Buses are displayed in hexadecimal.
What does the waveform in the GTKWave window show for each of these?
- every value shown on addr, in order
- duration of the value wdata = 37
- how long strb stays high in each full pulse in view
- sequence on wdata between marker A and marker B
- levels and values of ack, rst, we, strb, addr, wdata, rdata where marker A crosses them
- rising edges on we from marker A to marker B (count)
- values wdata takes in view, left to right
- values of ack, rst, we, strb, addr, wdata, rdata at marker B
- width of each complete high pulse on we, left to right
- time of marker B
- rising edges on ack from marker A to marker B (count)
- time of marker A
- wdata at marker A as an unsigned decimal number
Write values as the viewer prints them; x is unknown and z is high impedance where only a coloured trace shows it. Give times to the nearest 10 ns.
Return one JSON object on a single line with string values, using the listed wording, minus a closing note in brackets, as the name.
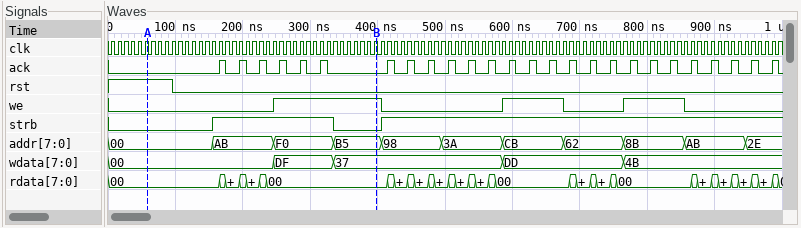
{"every value shown on addr, in order": "00, AB, F0, B5, 98, 3A, CB, 62, 8B, AB, 2E", "duration of the value wdata = 37": "250 ns", "how long strb stays high in each full pulse in view": "180 ns", "sequence on wdata between marker A and marker B": "00, DF, 37", "levels and values of ack, rst, we, strb, addr, wdata, rdata where marker A crosses them": "ack=0, rst=1, we=0, strb=0, addr=00, wdata=00, rdata=00", "rising edges on we from marker A to marker B": "1", "values wdata takes in view, left to right": "00, DF, 37, DD, 4B", "values of ack, rst, we, strb, addr, wdata, rdata at marker B": "ack=0, rst=0, we=1, strb=0, addr=B5, wdata=37, rdata=00", "width of each complete high pulse on we, left to right": "160 ns, 90 ns, 90 ns", "time of marker B": "400 ns", "rising edges on ack from marker A to marker B": "6", "time of marker A": "60 ns", "wdata at marker A as an unsigned decimal number": "0"}
